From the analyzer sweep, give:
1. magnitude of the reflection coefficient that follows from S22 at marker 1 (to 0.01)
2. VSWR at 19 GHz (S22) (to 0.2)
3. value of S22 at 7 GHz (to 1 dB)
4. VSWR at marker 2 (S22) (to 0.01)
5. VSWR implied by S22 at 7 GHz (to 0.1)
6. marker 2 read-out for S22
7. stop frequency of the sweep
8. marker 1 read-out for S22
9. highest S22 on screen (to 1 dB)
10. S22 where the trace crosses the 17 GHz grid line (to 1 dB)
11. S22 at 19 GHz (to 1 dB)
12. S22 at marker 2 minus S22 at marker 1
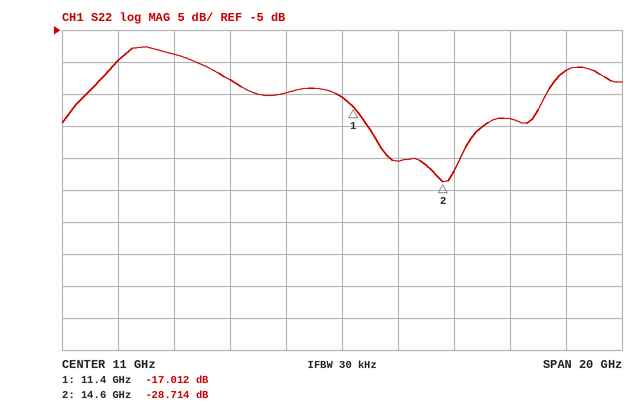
0.14
1.8
-13 dB
1.08
1.6
-28.714 dB
21 GHz
-17.012 dB
-8 dB
-19 dB
-11 dB
-11.702 dB
